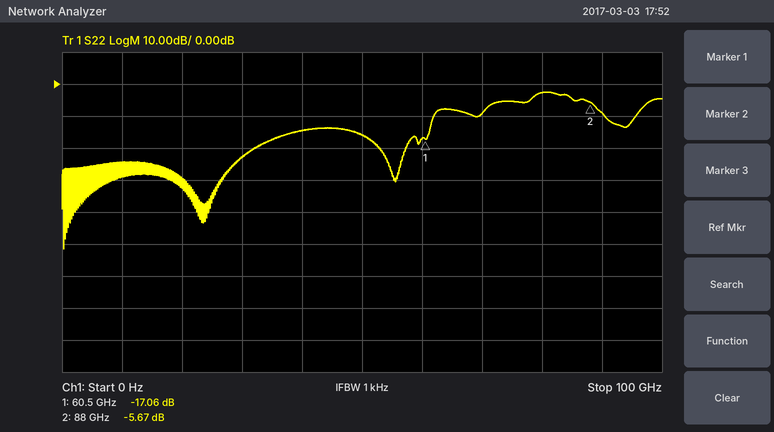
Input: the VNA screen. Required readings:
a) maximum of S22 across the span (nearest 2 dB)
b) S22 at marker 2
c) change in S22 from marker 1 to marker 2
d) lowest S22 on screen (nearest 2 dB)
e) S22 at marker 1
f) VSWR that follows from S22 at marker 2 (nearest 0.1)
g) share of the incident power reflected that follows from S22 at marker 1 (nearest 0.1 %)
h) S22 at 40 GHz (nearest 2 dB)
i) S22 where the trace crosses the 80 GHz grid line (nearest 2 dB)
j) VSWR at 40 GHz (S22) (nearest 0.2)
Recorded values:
-2 dB
-5.67 dB
11.39 dB
-52 dB
-17.06 dB
3.2
2.0 %
-14 dB
-2 dB
1.4
